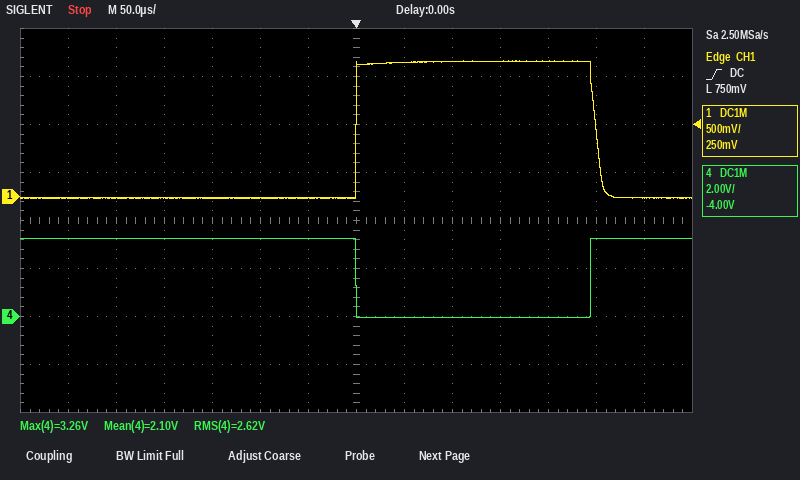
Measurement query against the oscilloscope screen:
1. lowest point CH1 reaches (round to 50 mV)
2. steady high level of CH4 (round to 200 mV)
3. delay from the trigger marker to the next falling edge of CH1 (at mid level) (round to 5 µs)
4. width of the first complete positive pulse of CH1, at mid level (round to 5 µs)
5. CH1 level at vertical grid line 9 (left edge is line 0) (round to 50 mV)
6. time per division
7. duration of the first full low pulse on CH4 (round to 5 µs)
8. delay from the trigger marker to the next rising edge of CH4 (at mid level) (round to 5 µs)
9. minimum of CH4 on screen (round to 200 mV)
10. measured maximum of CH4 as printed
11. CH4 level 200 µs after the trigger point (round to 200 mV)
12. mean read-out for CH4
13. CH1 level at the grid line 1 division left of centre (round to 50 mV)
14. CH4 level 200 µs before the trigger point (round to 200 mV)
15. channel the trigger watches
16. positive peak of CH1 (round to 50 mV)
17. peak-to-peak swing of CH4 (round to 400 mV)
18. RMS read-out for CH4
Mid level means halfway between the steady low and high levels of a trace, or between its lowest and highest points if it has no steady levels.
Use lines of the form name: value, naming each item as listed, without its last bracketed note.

lowest point CH1 reaches: 0 mV
steady high level of CH4: 3.2 V
delay from the trigger marker to the next falling edge of CH1 (at mid level): 250 µs
width of the first complete positive pulse of CH1, at mid level: 250 µs
CH1 level at vertical grid line 9 (left edge is line 0): 1.40 V
time per division: 50 µs
duration of the first full low pulse on CH4: 245 µs
delay from the trigger marker to the next rising edge of CH4 (at mid level): 245 µs
minimum of CH4 on screen: 0.0 V
measured maximum of CH4 as printed: 3.26 V
CH4 level 200 µs after the trigger point: 0.0 V
mean read-out for CH4: 2.10 V
CH1 level at the grid line 1 division left of centre: 0 mV
CH4 level 200 µs before the trigger point: 3.2 V
channel the trigger watches: CH1
positive peak of CH1: 1.40 V
peak-to-peak swing of CH4: 3.2 V
RMS read-out for CH4: 2.62 V
